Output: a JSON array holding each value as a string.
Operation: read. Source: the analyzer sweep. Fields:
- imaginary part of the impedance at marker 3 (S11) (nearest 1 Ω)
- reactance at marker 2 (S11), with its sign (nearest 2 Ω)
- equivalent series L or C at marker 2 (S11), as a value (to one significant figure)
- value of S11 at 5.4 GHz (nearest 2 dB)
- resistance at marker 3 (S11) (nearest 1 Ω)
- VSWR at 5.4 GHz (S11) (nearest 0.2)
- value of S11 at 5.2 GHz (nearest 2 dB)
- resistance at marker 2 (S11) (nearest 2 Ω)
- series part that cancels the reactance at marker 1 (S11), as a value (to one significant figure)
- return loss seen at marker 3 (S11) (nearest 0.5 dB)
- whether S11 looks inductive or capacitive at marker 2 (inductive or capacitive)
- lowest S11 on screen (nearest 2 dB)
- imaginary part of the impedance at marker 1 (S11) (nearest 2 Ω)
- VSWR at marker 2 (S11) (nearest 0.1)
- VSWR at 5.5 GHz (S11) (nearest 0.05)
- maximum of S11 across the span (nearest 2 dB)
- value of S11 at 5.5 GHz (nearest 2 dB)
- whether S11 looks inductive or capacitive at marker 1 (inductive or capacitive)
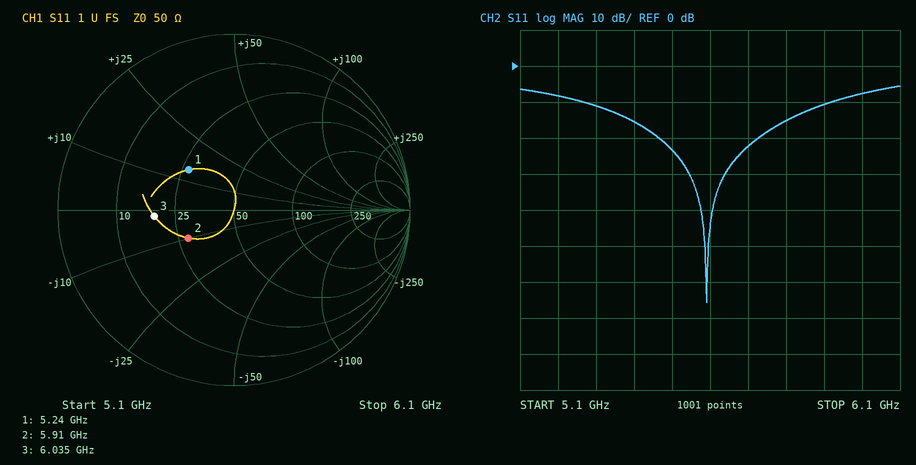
["-2 Ω", "-10 Ω", "3 pF", "-16 dB", "19 Ω", "1.4", "-8 dB", "28 Ω", "2 pF", "7.0 dB", "capacitive", "-66 dB", "+14 Ω", "1.9", "1.15", "-6 dB", "-24 dB", "inductive"]
